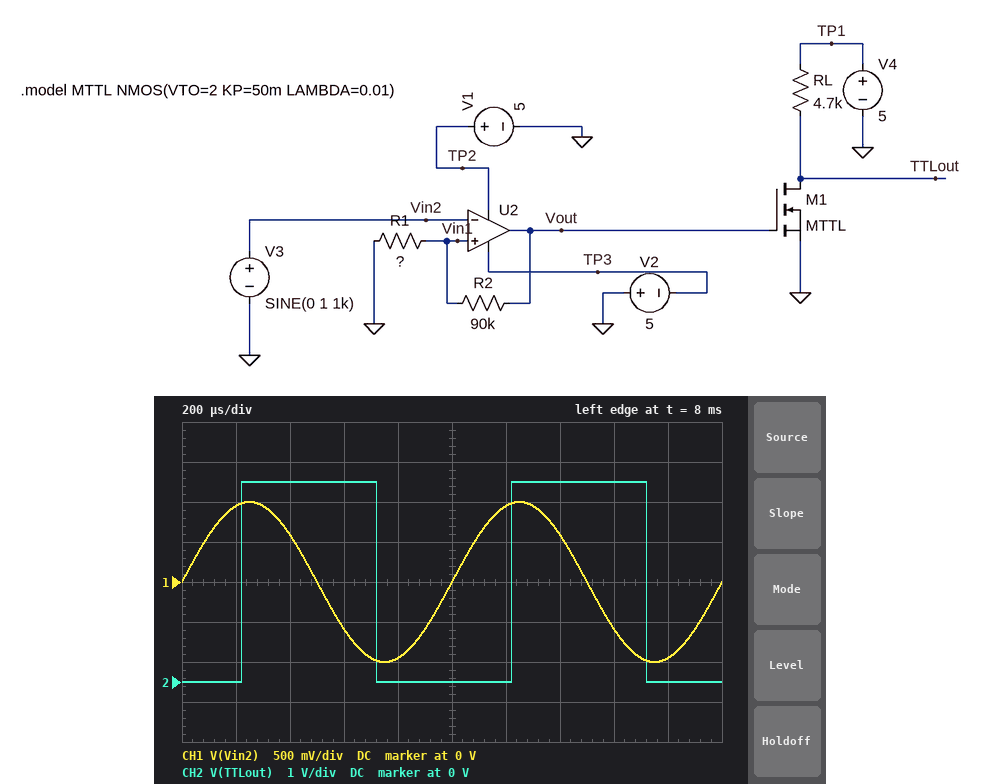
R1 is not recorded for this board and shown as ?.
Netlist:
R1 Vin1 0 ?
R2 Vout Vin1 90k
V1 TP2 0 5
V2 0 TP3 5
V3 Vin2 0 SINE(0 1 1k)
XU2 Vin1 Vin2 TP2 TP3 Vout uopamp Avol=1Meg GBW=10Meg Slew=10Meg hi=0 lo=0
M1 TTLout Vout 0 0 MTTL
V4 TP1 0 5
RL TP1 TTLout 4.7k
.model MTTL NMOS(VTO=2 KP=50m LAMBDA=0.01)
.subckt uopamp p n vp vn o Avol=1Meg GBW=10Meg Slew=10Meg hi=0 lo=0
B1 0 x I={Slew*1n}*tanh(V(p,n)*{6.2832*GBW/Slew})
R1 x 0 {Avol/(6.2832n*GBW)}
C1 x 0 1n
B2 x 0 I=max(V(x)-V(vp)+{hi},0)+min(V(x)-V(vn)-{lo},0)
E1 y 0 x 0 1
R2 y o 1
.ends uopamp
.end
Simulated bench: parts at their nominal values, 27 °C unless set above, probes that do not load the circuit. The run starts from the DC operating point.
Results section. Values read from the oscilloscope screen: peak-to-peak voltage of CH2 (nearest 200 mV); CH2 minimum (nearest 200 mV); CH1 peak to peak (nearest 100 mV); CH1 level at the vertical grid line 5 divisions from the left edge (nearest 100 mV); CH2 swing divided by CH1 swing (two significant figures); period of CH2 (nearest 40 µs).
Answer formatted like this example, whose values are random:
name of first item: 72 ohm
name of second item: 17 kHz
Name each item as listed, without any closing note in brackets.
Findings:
peak-to-peak voltage of CH2: 5.0 V
CH2 minimum: 0 V
CH1 peak to peak: 2.0 V
CH1 level at the vertical grid line 5 divisions from the left edge: 0 V
CH2 swing divided by CH1 swing: 2.5
period of CH2: 1.00 ms
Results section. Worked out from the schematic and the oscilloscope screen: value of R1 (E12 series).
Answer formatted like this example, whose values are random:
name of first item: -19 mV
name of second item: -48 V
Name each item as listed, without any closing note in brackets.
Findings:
value of R1: 22 kΩ
